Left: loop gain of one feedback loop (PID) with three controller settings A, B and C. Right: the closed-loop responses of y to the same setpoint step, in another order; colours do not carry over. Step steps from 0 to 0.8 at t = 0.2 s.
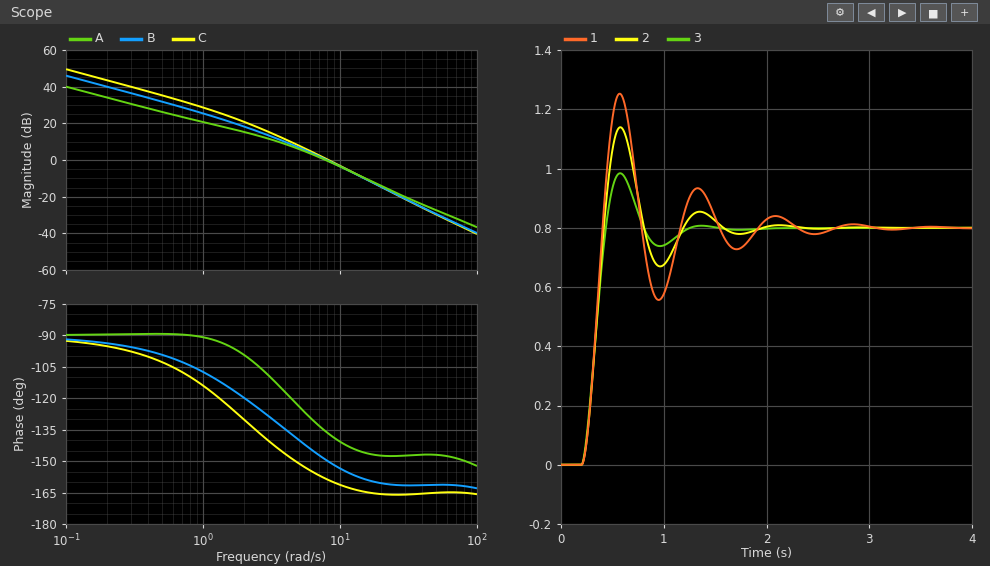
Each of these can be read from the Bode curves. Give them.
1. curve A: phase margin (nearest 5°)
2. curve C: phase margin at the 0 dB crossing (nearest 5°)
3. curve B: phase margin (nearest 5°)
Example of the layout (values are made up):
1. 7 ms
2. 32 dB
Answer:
1. 45°
2. 20°
3. 30°
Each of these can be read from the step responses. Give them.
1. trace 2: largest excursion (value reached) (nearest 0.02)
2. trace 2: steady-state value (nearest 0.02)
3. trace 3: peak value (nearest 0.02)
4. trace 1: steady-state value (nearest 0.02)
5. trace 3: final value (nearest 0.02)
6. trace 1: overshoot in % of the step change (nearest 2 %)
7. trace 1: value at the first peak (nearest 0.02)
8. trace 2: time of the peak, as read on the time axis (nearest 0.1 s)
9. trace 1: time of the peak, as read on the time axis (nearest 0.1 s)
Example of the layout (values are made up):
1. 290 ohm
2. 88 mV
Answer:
1. 1.14
2. 0.80
3. 0.98
4. 0.80
5. 0.80
6. 56 %
7. 1.26
8. 0.6 s
9. 0.6 s
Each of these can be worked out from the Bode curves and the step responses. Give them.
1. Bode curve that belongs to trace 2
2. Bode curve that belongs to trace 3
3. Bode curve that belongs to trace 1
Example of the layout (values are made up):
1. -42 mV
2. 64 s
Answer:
1. B
2. A
3. C
